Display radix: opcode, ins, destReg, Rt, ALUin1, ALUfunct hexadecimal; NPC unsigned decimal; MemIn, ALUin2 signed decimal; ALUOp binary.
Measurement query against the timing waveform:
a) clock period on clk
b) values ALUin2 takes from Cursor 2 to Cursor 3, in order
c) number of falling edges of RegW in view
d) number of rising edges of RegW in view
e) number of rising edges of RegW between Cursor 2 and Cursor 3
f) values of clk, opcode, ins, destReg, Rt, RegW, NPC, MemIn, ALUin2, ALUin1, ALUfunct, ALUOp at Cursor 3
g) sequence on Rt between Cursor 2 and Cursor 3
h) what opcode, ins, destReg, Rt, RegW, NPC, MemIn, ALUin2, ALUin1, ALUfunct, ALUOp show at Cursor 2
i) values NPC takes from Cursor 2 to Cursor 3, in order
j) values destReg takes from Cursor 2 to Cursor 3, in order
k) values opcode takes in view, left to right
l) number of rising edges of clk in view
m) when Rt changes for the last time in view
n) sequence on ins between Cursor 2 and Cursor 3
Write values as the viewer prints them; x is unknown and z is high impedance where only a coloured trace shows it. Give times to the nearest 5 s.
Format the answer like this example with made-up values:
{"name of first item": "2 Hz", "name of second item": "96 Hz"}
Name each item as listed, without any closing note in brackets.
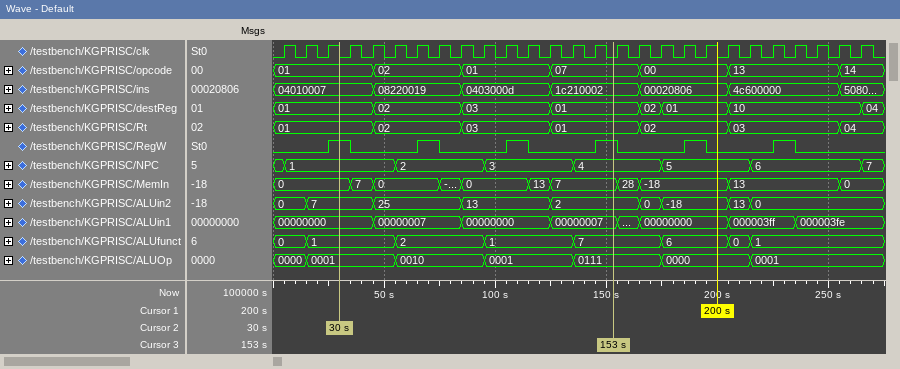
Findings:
{"clock period on clk": "10 s", "values ALUin2 takes from Cursor 2 to Cursor 3, in order": "7, 25, 13, 2", "number of falling edges of RegW in view": "6", "number of rising edges of RegW in view": "6", "number of rising edges of RegW between Cursor 2 and Cursor 3": "3", "values of clk, opcode, ins, destReg, Rt, RegW, NPC, MemIn, ALUin2, ALUin1, ALUfunct, ALUOp at Cursor 3": "clk=0, opcode=07, ins=1c210002, destReg=01, Rt=01, RegW=1, NPC=4, MemIn=7, ALUin2=2, ALUin1=00000007, ALUfunct=7, ALUOp=0111", "sequence on Rt between Cursor 2 and Cursor 3": "01, 02, 03, 01", "what opcode, ins, destReg, Rt, RegW, NPC, MemIn, ALUin2, ALUin1, ALUfunct, ALUOp show at Cursor 2": "opcode=01, ins=04010007, destReg=01, Rt=01, RegW=1, NPC=1, MemIn=0, ALUin2=7, ALUin1=00000000, ALUfunct=1, ALUOp=0001", "values NPC takes from Cursor 2 to Cursor 3, in order": "1, 2, 3, 4", "values destReg takes from Cursor 2 to Cursor 3, in order": "01, 02, 03, 01", "values opcode takes in view, left to right": "01, 02, 01, 07, 00, 13, 14", "number of rising edges of clk in view": "27", "when Rt changes for the last time in view": "255 s", "sequence on ins between Cursor 2 and Cursor 3": "04010007, 08220019, 0403000d, 1c210002"}
